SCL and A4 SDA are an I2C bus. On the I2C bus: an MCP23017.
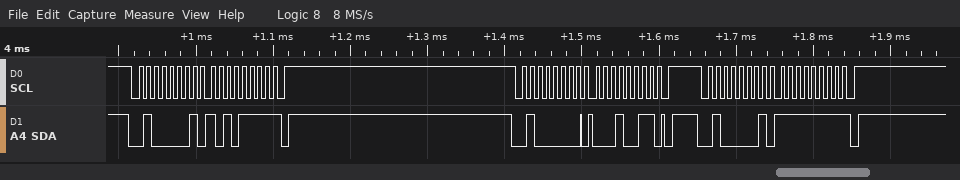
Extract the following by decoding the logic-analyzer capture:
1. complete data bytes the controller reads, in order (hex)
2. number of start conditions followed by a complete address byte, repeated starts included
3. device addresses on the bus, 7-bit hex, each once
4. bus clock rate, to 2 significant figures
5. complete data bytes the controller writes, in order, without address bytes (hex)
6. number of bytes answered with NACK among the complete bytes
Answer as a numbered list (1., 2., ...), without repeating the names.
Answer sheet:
1. AF FF
2. 3
3. 0x20
4. 100 kHz
5. 13
6. 2
